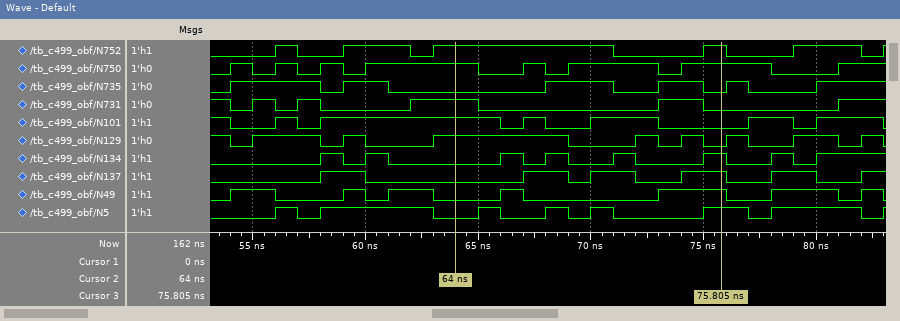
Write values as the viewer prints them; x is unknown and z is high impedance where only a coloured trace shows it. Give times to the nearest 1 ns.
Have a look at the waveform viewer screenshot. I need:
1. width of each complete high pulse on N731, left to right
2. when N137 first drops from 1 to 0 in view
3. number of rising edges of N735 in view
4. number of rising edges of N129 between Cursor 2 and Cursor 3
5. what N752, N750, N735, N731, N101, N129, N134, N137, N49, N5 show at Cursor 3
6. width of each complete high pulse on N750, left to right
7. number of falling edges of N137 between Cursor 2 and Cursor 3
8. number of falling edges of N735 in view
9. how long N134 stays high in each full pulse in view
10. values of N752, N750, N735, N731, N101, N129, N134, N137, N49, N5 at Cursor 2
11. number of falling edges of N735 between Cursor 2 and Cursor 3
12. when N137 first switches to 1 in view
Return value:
1 ns, 1 ns, 3 ns, 2 ns
60 ns
6
2
N752=1, N750=1, N735=0, N731=0, N101=0, N129=0, N134=1, N137=1, N49=1, N5=1
1 ns, 1 ns, 1 ns, 5 ns, 1 ns, 4 ns, 4 ns
2
5
1 ns, 1 ns, 1 ns, 1 ns, 1 ns, 1 ns, 1 ns
N752=1, N750=1, N735=0, N731=1, N101=1, N129=1, N134=0, N137=0, N49=0, N5=0
2
58 ns
